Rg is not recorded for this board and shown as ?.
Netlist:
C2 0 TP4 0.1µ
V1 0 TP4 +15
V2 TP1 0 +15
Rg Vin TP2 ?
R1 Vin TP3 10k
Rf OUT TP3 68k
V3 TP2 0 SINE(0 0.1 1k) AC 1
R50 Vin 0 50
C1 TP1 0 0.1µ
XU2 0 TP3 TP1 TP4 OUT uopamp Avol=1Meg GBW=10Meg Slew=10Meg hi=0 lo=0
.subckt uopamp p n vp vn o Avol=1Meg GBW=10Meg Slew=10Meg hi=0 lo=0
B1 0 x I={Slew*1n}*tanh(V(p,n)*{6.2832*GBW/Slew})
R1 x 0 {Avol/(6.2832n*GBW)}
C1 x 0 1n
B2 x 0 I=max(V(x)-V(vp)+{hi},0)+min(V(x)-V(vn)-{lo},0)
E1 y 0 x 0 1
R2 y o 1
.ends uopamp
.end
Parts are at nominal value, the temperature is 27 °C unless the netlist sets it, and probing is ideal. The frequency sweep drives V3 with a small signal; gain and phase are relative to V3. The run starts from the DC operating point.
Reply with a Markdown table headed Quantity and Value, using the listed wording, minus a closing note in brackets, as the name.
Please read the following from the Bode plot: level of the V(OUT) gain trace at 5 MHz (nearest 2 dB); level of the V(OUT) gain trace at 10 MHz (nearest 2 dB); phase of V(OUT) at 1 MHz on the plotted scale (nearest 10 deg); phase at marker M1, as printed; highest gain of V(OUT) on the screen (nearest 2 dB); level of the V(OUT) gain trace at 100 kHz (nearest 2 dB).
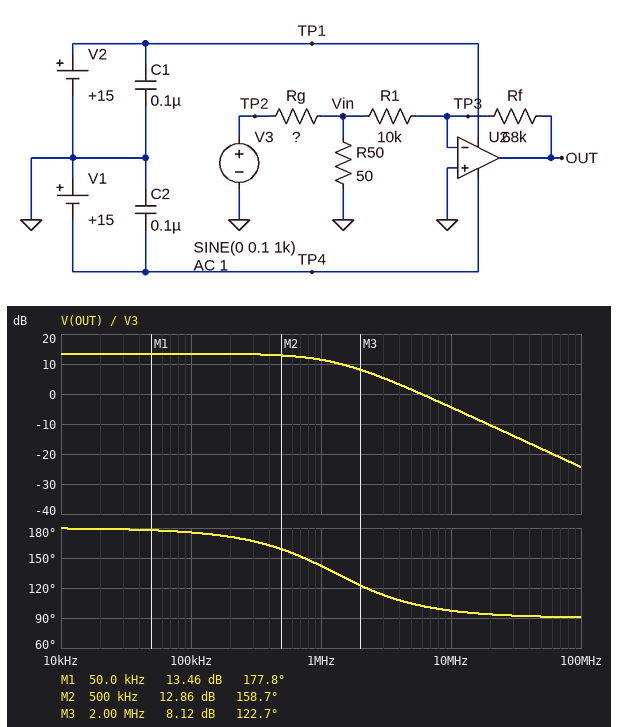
| Quantity | Value |
|---|---|
| level of the V(OUT) gain trace at 5 MHz | 2 dB |
| level of the V(OUT) gain trace at 10 MHz | -4 dB |
| phase of V(OUT) at 1 MHz on the plotted scale | 140 deg |
| phase at marker M1, as printed | 177.8 deg |
| highest gain of V(OUT) on the screen | 14 dB |
| level of the V(OUT) gain trace at 100 kHz | 14 dB |
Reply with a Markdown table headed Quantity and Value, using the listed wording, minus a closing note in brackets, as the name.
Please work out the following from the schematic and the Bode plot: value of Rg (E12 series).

| Quantity | Value |
|---|---|
| value of Rg | 22 Ω |
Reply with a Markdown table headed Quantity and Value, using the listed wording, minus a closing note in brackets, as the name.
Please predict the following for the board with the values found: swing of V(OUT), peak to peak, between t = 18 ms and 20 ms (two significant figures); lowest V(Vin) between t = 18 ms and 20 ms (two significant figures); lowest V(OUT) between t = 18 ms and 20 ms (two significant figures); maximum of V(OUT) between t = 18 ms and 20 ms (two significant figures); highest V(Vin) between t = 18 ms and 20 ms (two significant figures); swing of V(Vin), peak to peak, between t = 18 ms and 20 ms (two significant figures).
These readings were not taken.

| Quantity | Value |
|---|---|
| swing of V(OUT), peak to peak, between t = 18 ms and 20 ms | 940 mV |
| lowest V(Vin) between t = 18 ms and 20 ms | -69 mV |
| lowest V(OUT) between t = 18 ms and 20 ms | -470 mV |
| maximum of V(OUT) between t = 18 ms and 20 ms | 470 mV |
| highest V(Vin) between t = 18 ms and 20 ms | 69 mV |
| swing of V(Vin), peak to peak, between t = 18 ms and 20 ms | 140 mV |
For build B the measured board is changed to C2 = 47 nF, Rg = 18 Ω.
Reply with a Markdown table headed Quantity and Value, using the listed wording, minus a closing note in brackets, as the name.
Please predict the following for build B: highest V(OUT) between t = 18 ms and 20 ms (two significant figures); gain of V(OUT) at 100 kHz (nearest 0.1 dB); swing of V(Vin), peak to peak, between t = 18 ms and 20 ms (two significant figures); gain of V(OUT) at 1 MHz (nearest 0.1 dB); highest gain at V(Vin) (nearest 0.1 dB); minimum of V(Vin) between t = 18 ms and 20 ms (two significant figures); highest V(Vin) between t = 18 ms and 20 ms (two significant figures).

| Quantity | Value |
|---|---|
| highest V(OUT) between t = 18 ms and 20 ms | 500 mV |
| gain of V(OUT) at 100 kHz | 13.9 dB |
| swing of V(Vin), peak to peak, between t = 18 ms and 20 ms | 150 mV |
| gain of V(OUT) at 1 MHz | 11.9 dB |
| highest gain at V(Vin) | -2.7 dB |
| minimum of V(Vin) between t = 18 ms and 20 ms | -73 mV |
| highest V(Vin) between t = 18 ms and 20 ms | 73 mV |
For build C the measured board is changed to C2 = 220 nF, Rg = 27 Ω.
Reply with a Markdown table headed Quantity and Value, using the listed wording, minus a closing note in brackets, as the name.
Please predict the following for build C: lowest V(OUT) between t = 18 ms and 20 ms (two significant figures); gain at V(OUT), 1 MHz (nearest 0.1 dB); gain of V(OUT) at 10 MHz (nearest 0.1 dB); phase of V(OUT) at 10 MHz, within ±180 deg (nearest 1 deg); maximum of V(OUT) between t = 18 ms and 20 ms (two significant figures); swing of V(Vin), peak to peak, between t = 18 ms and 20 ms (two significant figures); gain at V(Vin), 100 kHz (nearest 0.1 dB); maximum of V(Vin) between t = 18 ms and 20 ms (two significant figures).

| Quantity | Value |
|---|---|
| lowest V(OUT) between t = 18 ms and 20 ms | -440 mV |
| gain at V(OUT), 1 MHz | 10.8 dB |
| gain of V(OUT) at 10 MHz | -5.0 dB |
| phase of V(OUT) at 10 MHz, within ±180 deg | 97 deg |
| maximum of V(OUT) between t = 18 ms and 20 ms | 440 mV |
| swing of V(Vin), peak to peak, between t = 18 ms and 20 ms | 130 mV |
| gain at V(Vin), 100 kHz | -3.8 dB |
| maximum of V(Vin) between t = 18 ms and 20 ms | 65 mV |
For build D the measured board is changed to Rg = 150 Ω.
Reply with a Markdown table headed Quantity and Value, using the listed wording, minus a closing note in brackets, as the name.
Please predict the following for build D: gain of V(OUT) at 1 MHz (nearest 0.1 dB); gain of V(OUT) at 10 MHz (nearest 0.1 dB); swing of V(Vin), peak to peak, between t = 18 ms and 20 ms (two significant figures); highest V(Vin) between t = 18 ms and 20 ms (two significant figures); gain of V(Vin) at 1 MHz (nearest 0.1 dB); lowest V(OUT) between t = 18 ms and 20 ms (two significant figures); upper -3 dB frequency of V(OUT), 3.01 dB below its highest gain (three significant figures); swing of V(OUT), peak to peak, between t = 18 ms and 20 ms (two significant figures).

| Quantity | Value |
|---|---|
| gain of V(OUT) at 1 MHz | 2.5 dB |
| gain of V(OUT) at 10 MHz | -13.3 dB |
| swing of V(Vin), peak to peak, between t = 18 ms and 20 ms | 50 mV |
| highest V(Vin) between t = 18 ms and 20 ms | 25 mV |
| gain of V(Vin) at 1 MHz | -12.1 dB |
| lowest V(OUT) between t = 18 ms and 20 ms | -170 mV |
| upper -3 dB frequency of V(OUT), 3.01 dB below its highest gain | 1.29 MHz |
| swing of V(OUT), peak to peak, between t = 18 ms and 20 ms | 340 mV |
